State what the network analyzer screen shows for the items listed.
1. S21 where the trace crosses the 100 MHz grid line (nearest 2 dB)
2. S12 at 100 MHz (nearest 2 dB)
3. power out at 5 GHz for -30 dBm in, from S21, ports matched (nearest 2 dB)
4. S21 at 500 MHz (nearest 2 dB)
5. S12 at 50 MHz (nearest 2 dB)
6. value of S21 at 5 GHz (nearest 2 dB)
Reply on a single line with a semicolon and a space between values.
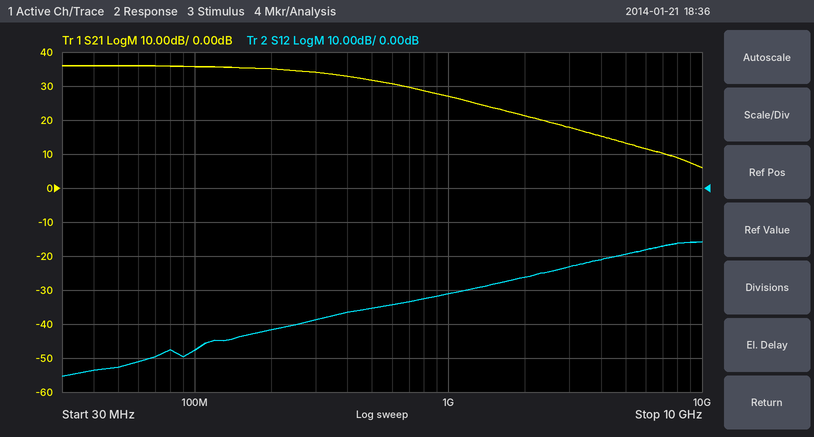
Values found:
36 dB; -48 dB; -16 dBm; 32 dB; -52 dB; 14 dB
